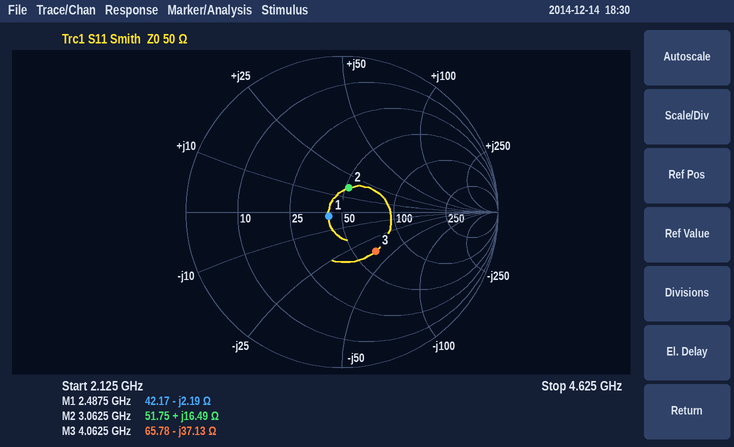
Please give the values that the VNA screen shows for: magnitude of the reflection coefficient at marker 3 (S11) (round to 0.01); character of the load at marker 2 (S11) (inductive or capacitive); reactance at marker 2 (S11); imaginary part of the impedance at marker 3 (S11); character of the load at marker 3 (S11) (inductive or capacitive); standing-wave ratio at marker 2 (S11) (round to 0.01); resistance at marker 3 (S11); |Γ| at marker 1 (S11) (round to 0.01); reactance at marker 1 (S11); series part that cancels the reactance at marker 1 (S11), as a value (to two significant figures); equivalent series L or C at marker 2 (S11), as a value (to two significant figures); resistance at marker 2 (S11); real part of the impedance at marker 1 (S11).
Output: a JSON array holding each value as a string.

["0.33", "inductive", "+16.49 Ω", "-37.13 Ω", "capacitive", "1.38", "65.78 Ω", "0.09", "-2.19 Ω", "140 pH", "860 pH", "51.75 Ω", "42.17 Ω"]
